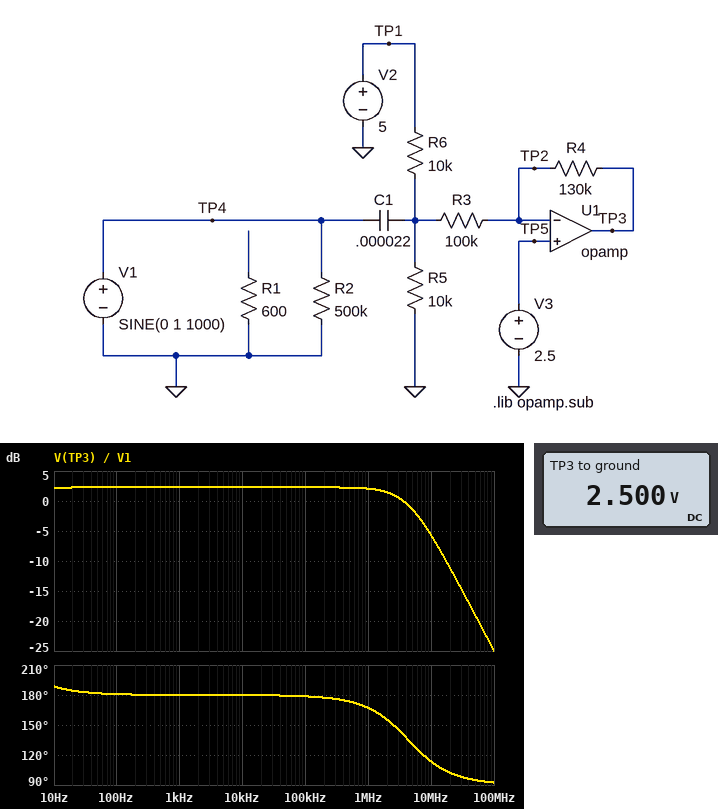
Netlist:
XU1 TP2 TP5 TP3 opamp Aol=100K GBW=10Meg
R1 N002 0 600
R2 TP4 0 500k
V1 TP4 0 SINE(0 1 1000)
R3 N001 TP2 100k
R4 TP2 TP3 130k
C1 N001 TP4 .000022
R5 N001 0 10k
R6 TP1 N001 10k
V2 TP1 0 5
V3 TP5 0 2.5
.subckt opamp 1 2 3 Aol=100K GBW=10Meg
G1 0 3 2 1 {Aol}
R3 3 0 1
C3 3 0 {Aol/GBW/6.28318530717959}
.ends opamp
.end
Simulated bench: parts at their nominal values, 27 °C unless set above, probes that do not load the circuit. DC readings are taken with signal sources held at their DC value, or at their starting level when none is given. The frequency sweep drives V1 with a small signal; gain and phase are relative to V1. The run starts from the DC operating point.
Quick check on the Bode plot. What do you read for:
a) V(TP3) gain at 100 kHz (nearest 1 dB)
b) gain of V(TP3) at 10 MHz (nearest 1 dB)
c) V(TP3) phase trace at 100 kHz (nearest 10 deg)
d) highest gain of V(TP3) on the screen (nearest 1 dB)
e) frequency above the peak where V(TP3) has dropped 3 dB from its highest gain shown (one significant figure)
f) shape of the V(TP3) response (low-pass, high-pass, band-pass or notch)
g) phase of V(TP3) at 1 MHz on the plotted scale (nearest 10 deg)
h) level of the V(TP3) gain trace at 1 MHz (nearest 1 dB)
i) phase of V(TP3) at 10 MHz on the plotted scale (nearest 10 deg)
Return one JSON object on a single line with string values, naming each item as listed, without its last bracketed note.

{"V(TP3) gain at 100 kHz": "2 dB", "gain of V(TP3) at 10 MHz": "-6 dB", "V(TP3) phase trace at 100 kHz": "180 deg", "highest gain of V(TP3) on the screen": "2 dB", "frequency above the peak where V(TP3) has dropped 3 dB from its highest gain shown": "4 MHz", "shape of the V(TP3) response": "low-pass", "phase of V(TP3) at 1 MHz on the plotted scale": "170 deg", "level of the V(TP3) gain trace at 1 MHz": "2 dB", "phase of V(TP3) at 10 MHz on the plotted scale": "110 deg"}
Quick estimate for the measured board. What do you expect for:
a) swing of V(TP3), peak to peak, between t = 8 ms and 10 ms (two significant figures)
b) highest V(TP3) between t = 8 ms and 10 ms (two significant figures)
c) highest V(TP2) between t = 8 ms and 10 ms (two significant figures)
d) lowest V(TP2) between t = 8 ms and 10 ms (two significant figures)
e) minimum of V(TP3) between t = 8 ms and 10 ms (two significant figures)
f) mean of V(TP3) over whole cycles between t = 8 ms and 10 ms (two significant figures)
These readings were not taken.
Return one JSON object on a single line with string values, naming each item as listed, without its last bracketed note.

{"swing of V(TP3), peak to peak, between t = 8 ms and 10 ms": "2.6 V", "highest V(TP3) between t = 8 ms and 10 ms": "3.8 V", "highest V(TP2) between t = 8 ms and 10 ms": "2.5 V", "lowest V(TP2) between t = 8 ms and 10 ms": "2.5 V", "minimum of V(TP3) between t = 8 ms and 10 ms": "1.2 V", "mean of V(TP3) over whole cycles between t = 8 ms and 10 ms": "2.5 V"}
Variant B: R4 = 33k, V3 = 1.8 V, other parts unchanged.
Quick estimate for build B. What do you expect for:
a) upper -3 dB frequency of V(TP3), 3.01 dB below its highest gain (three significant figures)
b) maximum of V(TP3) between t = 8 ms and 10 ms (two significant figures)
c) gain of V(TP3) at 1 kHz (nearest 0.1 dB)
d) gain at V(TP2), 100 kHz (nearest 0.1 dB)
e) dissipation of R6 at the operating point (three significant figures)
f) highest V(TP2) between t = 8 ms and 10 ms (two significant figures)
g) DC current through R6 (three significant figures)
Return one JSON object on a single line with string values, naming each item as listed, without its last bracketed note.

{"upper -3 dB frequency of V(TP3), 3.01 dB below its highest gain": "7.52 MHz", "maximum of V(TP3) between t = 8 ms and 10 ms": "1.9 V", "gain of V(TP3) at 1 kHz": "-9.6 dB", "gain at V(TP2), 100 kHz": "-49.6 dB", "dissipation of R6 at the operating point": "642 µW", "highest V(TP2) between t = 8 ms and 10 ms": "1.8 V", "DC current through R6": "253 µA"}
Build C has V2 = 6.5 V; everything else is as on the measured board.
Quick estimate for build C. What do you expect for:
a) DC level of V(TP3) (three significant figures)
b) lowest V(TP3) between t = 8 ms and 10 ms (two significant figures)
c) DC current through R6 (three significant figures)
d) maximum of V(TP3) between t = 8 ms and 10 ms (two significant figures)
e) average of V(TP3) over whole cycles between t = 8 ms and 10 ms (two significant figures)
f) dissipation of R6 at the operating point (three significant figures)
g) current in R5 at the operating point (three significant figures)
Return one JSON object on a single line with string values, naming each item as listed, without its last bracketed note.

{"DC level of V(TP3)": "1.57 V", "lowest V(TP3) between t = 8 ms and 10 ms": "270 mV", "DC current through R6": "329 µA", "maximum of V(TP3) between t = 8 ms and 10 ms": "2.9 V", "average of V(TP3) over whole cycles between t = 8 ms and 10 ms": "1.6 V", "dissipation of R6 at the operating point": "1.08 mW", "current in R5 at the operating point": "321 µA"}
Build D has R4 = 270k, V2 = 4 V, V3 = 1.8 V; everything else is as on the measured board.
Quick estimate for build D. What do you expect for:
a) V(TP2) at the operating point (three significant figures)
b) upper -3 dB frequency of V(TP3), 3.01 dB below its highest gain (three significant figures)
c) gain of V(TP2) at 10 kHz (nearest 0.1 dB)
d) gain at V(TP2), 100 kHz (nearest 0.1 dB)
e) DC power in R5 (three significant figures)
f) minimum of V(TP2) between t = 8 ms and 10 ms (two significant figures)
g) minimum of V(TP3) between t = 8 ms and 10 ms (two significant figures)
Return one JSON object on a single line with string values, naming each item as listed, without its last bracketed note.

{"V(TP2) at the operating point": "1.80 V", "upper -3 dB frequency of V(TP3), 3.01 dB below its highest gain": "2.70 MHz", "gain of V(TP2) at 10 kHz": "-51.4 dB", "gain at V(TP2), 100 kHz": "-31.4 dB", "DC power in R5": "396 µW", "minimum of V(TP2) between t = 8 ms and 10 ms": "1.8 V", "minimum of V(TP3) between t = 8 ms and 10 ms": "-1.4 V"}
